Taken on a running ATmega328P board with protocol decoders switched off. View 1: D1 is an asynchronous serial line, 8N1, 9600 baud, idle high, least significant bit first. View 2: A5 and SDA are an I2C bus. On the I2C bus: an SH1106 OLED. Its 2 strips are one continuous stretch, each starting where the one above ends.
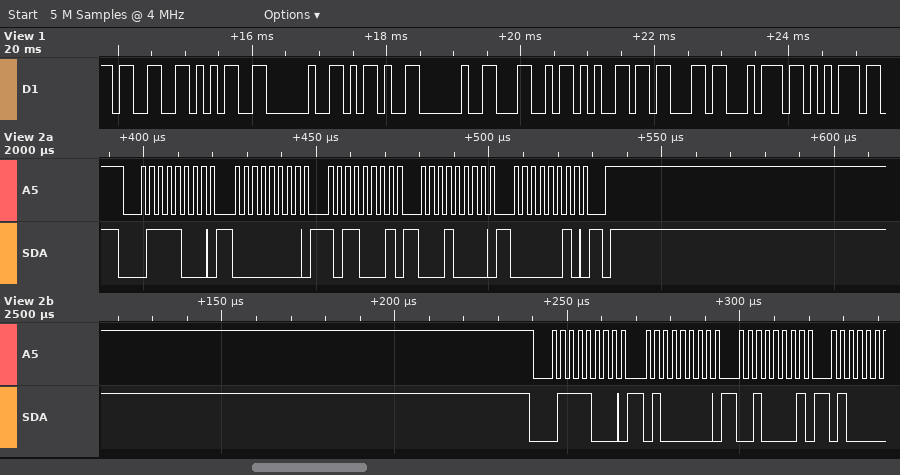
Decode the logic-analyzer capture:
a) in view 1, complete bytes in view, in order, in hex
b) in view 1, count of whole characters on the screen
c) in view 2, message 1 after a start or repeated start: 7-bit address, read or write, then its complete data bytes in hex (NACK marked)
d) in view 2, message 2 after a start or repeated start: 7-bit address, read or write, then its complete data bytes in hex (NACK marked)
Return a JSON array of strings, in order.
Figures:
["33 35 20 2D 20 4C 65 63 74 75", "10", "0x3C write: 00 B1 10 02", "0x3C write: 40 21"]
